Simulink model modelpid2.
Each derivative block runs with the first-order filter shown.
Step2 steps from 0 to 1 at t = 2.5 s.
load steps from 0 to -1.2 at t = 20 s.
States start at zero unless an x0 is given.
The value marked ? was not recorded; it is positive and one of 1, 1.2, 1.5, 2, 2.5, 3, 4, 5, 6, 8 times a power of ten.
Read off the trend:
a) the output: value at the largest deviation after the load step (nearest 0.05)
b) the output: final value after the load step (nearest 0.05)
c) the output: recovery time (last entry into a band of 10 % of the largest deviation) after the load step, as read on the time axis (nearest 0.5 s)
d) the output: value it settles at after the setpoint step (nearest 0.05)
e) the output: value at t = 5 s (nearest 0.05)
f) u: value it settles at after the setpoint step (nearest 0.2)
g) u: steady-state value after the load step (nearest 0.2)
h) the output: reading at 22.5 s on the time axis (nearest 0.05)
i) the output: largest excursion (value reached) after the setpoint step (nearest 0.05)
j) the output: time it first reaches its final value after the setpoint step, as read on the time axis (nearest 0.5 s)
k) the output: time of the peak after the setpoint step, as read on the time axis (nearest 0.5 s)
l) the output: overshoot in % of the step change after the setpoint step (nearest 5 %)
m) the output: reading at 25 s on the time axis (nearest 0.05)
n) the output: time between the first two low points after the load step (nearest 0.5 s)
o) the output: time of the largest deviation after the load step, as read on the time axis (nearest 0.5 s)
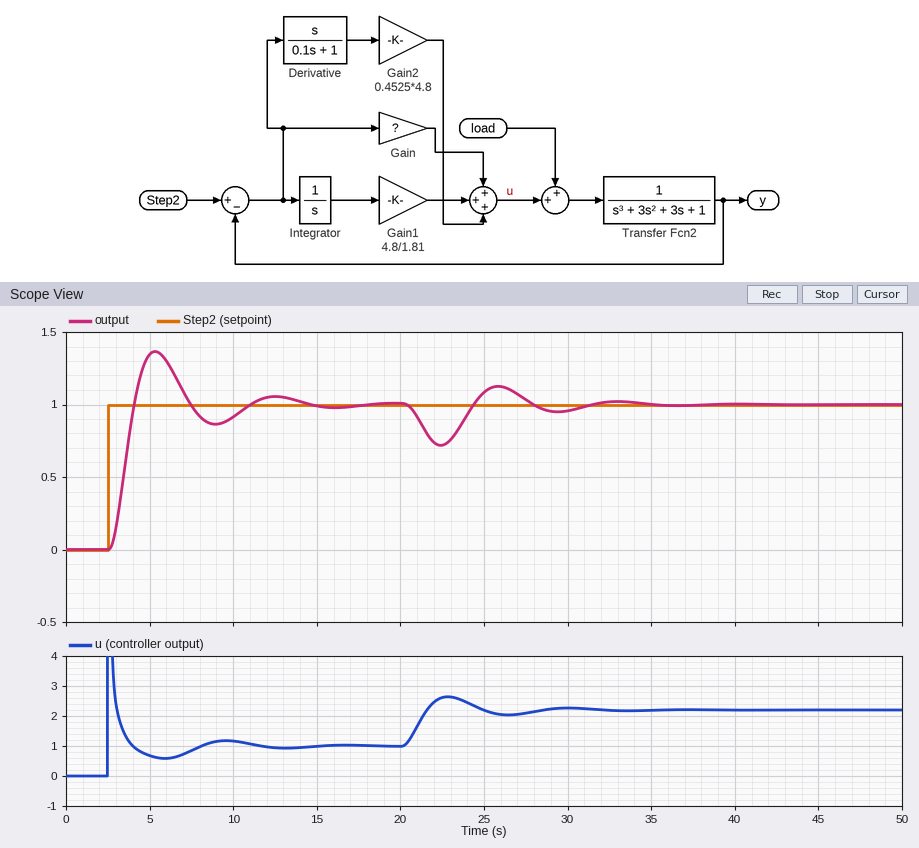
0.70
1.00
30.5 s
1.00
1.35
1.0
2.2
0.70
1.35
4.0 s
5.5 s
35 %
1.10
7.0 s
22.5 s
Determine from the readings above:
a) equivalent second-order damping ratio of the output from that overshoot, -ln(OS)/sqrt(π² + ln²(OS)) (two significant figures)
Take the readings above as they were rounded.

0.32
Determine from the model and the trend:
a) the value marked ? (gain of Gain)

2.5
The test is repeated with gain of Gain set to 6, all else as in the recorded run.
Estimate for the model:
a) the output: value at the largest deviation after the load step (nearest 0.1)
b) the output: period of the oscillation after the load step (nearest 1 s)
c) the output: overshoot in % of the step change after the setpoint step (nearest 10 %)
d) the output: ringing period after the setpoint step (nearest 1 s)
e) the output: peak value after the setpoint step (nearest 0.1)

0.8
4 s
50 %
4 s
1.5
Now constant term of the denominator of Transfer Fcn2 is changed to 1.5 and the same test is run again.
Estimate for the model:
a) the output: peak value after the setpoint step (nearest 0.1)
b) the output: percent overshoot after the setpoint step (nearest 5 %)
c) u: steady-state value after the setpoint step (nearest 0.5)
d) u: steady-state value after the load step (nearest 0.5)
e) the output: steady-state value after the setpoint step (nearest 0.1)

1.3
25 %
1.5
2.5
1.0
